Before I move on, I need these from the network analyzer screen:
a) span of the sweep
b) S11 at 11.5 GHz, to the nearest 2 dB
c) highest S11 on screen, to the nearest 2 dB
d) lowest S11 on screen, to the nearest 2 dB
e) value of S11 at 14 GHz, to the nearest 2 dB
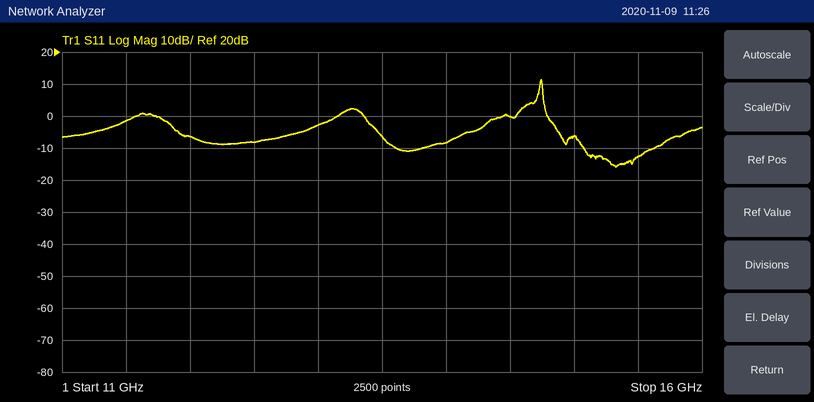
5 GHz
-2 dB
12 dB
-16 dB
-8 dB
